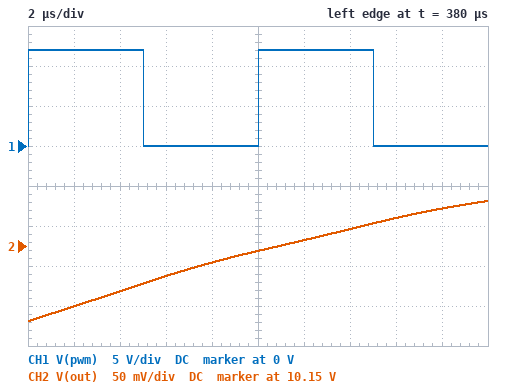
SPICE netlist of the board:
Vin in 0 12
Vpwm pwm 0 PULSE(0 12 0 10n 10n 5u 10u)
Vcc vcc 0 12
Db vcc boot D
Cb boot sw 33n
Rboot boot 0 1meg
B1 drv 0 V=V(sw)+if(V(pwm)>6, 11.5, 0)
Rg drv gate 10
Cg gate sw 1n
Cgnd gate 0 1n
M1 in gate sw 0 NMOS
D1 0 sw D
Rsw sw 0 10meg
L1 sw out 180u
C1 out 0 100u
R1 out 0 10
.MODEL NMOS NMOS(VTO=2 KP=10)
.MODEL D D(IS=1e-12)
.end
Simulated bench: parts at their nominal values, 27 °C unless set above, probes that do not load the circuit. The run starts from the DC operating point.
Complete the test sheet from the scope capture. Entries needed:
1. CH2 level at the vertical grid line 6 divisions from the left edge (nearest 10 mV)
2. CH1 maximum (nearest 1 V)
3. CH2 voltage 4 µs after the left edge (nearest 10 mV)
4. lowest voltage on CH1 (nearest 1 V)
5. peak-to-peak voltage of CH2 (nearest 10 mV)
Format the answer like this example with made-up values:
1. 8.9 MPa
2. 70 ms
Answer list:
1. 10.16 V
2. 12 V
3. 10.09 V
4. 0 V
5. 150 mV
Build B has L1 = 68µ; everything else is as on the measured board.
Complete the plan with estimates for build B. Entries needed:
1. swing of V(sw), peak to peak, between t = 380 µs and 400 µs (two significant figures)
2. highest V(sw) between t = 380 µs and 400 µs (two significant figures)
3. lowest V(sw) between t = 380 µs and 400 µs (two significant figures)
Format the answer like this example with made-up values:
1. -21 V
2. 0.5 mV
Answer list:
1. 17 V
2. 16 V
3. -680 mV
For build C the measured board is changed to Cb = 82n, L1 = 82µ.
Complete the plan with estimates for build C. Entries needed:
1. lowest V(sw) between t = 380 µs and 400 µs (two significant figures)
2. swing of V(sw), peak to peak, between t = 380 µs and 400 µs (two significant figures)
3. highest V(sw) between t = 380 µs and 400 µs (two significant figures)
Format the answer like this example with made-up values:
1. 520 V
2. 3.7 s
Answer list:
1. -680 mV
2. 17 V
3. 16 V
